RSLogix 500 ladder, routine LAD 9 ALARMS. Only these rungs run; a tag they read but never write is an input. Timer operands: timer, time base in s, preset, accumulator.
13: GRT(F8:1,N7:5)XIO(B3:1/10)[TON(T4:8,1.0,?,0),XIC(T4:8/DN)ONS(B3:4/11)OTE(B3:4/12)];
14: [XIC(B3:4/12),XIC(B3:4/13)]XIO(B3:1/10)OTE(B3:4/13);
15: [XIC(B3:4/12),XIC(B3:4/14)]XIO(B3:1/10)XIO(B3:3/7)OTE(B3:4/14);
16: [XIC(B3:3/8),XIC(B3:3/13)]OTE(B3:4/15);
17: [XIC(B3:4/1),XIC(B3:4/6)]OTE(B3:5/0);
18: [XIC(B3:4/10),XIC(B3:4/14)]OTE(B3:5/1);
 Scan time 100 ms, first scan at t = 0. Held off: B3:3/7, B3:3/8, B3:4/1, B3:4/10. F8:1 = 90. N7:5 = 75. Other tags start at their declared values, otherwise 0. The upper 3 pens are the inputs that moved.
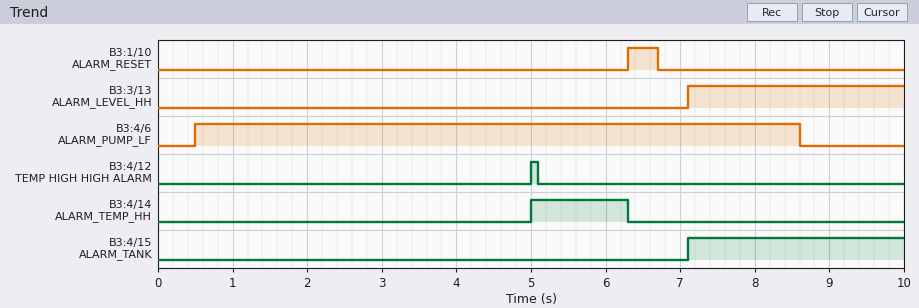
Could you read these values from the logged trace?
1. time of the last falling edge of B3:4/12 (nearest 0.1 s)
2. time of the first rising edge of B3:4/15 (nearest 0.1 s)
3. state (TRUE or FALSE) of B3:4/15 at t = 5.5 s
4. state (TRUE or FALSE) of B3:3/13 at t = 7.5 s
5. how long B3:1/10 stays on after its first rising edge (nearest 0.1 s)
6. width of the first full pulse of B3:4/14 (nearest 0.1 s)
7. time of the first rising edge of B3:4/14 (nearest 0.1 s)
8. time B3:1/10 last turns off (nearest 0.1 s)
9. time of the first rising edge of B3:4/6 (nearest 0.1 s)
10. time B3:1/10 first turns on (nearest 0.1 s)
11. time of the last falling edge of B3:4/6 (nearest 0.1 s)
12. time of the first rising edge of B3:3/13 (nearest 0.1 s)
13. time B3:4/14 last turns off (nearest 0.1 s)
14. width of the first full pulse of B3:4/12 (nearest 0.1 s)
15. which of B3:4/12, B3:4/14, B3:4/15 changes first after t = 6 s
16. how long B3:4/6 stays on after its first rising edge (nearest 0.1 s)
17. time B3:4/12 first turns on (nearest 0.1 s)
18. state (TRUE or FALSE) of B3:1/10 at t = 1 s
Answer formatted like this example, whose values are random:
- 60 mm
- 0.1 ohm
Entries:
- 5.1 s
- 7.1 s
- FALSE
- TRUE
- 0.4 s
- 1.3 s
- 5.0 s
- 6.7 s
- 0.5 s
- 6.3 s
- 8.6 s
- 7.1 s
- 6.3 s
- 0.1 s
- B3:4/14
- 8.1 s
- 5.0 s
- FALSE
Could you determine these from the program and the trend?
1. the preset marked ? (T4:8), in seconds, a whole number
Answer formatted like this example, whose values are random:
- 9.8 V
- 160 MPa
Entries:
- 5 s
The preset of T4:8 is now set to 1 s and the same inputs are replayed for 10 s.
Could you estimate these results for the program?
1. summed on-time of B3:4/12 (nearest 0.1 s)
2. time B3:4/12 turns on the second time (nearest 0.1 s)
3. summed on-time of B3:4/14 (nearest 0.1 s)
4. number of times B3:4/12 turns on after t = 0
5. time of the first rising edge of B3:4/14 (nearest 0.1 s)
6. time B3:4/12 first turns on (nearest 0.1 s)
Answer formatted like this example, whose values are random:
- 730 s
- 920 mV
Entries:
- 0.2 s
- 7.7 s
- 7.6 s
- 2
- 1.0 s
- 1.0 s
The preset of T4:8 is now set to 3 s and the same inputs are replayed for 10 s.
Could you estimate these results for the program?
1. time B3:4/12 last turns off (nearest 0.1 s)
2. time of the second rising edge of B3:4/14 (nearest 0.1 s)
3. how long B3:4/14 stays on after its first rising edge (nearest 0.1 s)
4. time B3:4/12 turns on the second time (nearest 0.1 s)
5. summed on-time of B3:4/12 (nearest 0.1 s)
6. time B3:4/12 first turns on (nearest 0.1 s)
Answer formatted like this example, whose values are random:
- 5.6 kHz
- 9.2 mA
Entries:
- 9.8 s
- 9.7 s
- 3.3 s
- 9.7 s
- 0.2 s
- 3.0 s
